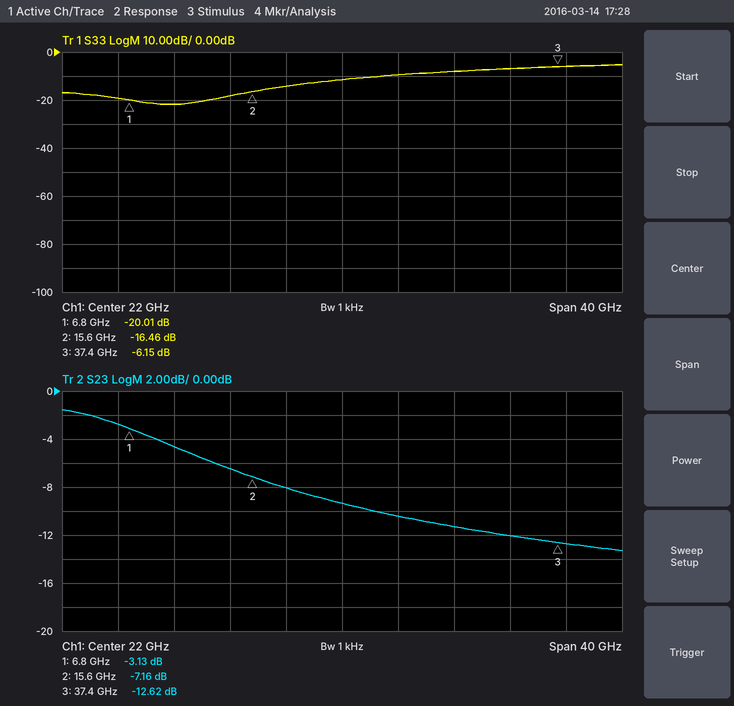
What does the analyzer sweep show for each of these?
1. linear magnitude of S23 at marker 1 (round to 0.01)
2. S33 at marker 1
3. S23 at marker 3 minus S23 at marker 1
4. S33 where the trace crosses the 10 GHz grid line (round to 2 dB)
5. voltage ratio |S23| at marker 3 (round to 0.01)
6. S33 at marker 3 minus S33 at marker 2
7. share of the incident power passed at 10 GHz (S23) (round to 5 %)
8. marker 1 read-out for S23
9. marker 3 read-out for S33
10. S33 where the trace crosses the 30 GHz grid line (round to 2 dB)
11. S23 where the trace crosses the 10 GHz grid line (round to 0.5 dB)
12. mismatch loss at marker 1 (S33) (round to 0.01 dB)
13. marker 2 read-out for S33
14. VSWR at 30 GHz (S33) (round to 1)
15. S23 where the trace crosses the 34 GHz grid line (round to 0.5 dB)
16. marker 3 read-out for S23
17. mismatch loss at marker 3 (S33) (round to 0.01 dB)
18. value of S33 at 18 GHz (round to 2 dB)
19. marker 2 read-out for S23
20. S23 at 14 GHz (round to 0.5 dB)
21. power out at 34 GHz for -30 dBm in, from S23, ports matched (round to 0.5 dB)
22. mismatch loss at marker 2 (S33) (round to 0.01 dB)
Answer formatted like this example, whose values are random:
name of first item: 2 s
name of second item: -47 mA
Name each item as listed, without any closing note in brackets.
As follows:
linear magnitude of S23 at marker 1: 0.70
S33 at marker 1: -20.01 dB
S23 at marker 3 minus S23 at marker 1: -9.49 dB
S33 where the trace crosses the 10 GHz grid line: -22 dB
voltage ratio |S23| at marker 3: 0.23
S33 at marker 3 minus S33 at marker 2: 10.31 dB
share of the incident power passed at 10 GHz (S23): 35 %
marker 1 read-out for S23: -3.13 dB
marker 3 read-out for S33: -6.15 dB
S33 where the trace crosses the 30 GHz grid line: -8 dB
S23 where the trace crosses the 10 GHz grid line: -4.5 dB
mismatch loss at marker 1 (S33): 0.04 dB
marker 2 read-out for S33: -16.46 dB
VSWR at 30 GHz (S33): 2
S23 where the trace crosses the 34 GHz grid line: -12.0 dB
marker 3 read-out for S23: -12.62 dB
mismatch loss at marker 3 (S33): 1.21 dB
value of S33 at 18 GHz: -14 dB
marker 2 read-out for S23: -7.16 dB
S23 at 14 GHz: -6.5 dB
power out at 34 GHz for -30 dBm in, from S23, ports matched: -42.0 dBm
mismatch loss at marker 2 (S33): 0.10 dB
